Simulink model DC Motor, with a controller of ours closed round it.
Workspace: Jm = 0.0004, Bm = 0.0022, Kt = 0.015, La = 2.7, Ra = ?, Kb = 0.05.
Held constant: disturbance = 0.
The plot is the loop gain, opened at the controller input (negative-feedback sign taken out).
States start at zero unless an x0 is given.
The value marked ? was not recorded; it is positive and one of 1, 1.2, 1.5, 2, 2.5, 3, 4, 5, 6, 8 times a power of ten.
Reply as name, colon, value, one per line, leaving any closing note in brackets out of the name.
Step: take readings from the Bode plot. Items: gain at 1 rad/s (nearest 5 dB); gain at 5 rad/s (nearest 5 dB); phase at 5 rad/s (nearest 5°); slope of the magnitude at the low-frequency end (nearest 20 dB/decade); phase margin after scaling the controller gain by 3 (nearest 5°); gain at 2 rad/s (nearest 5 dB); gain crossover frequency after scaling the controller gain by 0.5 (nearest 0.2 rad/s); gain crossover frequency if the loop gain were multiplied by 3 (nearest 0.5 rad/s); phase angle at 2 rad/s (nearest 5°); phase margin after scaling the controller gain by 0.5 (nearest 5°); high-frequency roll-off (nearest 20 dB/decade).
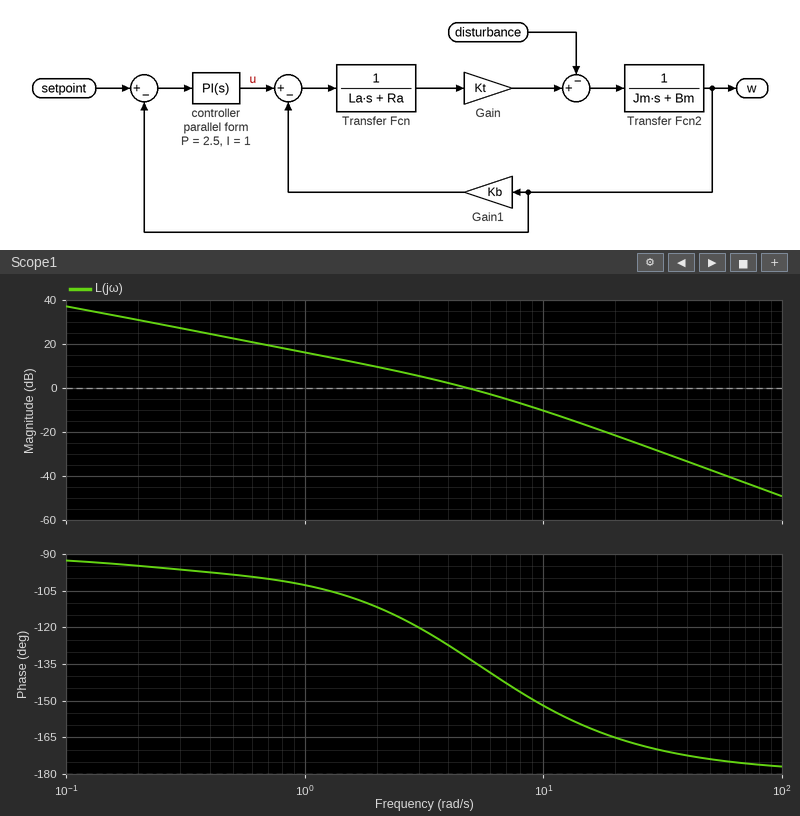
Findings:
gain at 1 rad/s: 15 dB
gain at 5 rad/s: 0 dB
phase at 5 rad/s: -135°
slope of the magnitude at the low-frequency end: -20 dB/decade
phase margin after scaling the controller gain by 3: 30°
gain at 2 rad/s: 10 dB
gain crossover frequency after scaling the controller gain by 0.5: 2.8 rad/s
gain crossover frequency if the loop gain were multiplied by 3: 9.5 rad/s
phase angle at 2 rad/s: -110°
phase margin after scaling the controller gain by 0.5: 60°
high-frequency roll-off: -40 dB/decade
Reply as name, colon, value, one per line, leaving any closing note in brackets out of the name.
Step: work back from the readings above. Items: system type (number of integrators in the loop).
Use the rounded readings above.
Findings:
system type: 1
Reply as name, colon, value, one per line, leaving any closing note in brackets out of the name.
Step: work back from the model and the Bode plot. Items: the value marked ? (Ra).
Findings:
the value marked ?: 0.6
